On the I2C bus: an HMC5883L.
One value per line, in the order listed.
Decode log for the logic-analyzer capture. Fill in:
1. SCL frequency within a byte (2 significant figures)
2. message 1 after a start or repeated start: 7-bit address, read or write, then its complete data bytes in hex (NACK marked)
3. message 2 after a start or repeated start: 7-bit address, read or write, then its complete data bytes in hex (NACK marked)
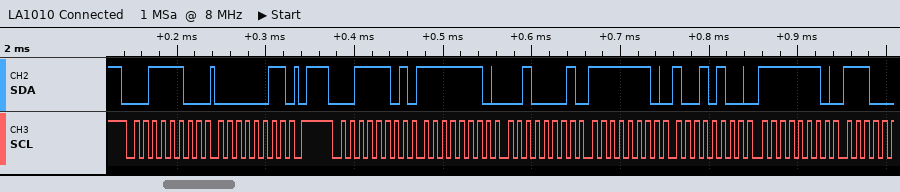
100 kHz
0x1E write: 03
0x1E read: FE 21 FE 94 FE
